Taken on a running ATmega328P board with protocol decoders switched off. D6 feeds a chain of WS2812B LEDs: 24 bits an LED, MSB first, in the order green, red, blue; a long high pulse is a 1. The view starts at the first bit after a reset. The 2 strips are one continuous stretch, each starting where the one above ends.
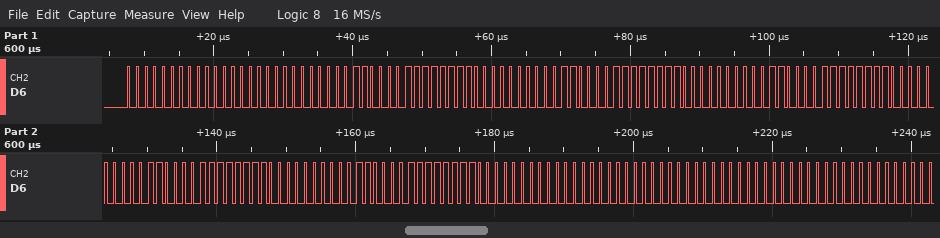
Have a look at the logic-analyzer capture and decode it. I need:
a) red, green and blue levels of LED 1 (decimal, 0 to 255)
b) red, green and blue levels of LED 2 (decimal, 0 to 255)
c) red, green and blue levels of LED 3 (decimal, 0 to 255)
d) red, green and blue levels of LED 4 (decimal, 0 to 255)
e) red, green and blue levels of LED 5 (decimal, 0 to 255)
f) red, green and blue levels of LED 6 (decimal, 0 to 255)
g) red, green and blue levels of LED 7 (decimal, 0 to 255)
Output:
0, 0, 0
255, 48, 0
255, 48, 0
255, 48, 0
255, 48, 0
255, 48, 0
0, 0, 0
